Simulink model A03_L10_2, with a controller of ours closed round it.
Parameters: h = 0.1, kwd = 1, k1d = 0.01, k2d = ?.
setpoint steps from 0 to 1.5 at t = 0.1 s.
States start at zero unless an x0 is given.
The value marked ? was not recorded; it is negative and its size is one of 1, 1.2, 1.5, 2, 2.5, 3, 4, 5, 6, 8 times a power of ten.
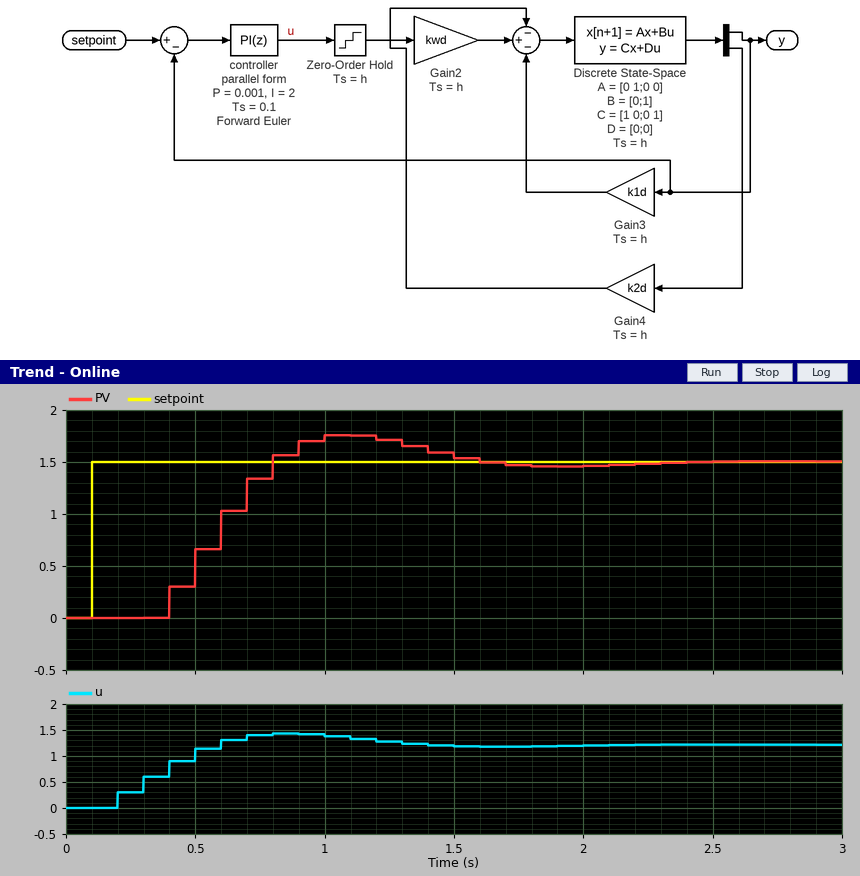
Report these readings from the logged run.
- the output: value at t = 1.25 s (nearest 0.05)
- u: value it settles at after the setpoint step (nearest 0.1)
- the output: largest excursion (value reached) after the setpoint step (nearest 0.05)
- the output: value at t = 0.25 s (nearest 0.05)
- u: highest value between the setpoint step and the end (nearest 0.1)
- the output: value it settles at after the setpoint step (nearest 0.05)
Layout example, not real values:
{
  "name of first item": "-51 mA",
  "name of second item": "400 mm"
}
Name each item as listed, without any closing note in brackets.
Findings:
{
  "the output: value at t = 1.25 s": "1.70",
  "u: value it settles at after the setpoint step": "1.2",
  "the output: largest excursion (value reached) after the setpoint step": "1.75",
  "the output: value at t = 0.25 s": "0.00",
  "u: highest value between the setpoint step and the end": "1.4",
  "the output: value it settles at after the setpoint step": "1.50"
}
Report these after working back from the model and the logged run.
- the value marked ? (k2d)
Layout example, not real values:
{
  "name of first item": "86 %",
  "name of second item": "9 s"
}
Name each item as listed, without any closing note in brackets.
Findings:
{
  "the value marked ?": "-0.2"
}
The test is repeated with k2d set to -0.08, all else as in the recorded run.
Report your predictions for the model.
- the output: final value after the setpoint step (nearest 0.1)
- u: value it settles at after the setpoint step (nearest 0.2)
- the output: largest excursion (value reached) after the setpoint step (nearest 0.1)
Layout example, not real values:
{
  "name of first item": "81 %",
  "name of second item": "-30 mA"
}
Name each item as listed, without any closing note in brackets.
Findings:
{
  "the output: final value after the setpoint step": "1.5",
  "u: value it settles at after the setpoint step": "1.4",
  "the output: largest excursion (value reached) after the setpoint step": "1.6"
}
